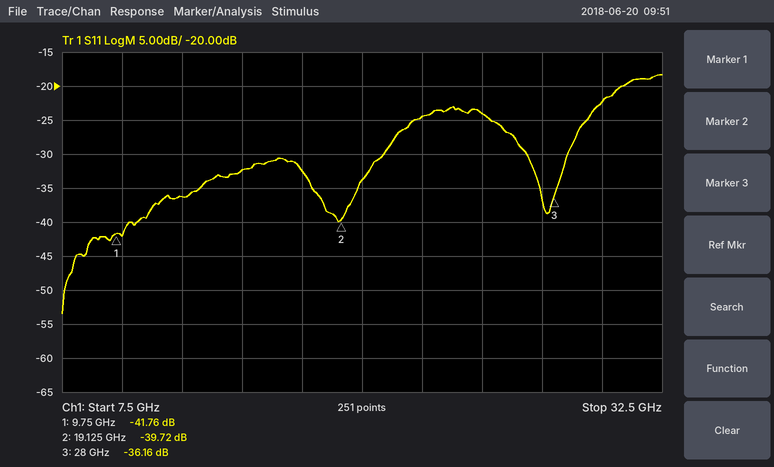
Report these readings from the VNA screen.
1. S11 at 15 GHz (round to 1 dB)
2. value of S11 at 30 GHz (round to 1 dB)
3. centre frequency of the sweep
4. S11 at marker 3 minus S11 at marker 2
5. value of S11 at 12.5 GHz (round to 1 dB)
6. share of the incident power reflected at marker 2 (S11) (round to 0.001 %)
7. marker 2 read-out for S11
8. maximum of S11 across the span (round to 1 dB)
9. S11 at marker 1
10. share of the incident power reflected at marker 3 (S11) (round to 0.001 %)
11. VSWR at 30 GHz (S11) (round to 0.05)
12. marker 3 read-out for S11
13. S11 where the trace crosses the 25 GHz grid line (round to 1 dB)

-32 dB
-22 dB
20 GHz
3.56 dB
-36 dB
0.011 %
-39.72 dB
-18 dB
-41.76 dB
0.024 %
1.15
-36.16 dB
-24 dB
